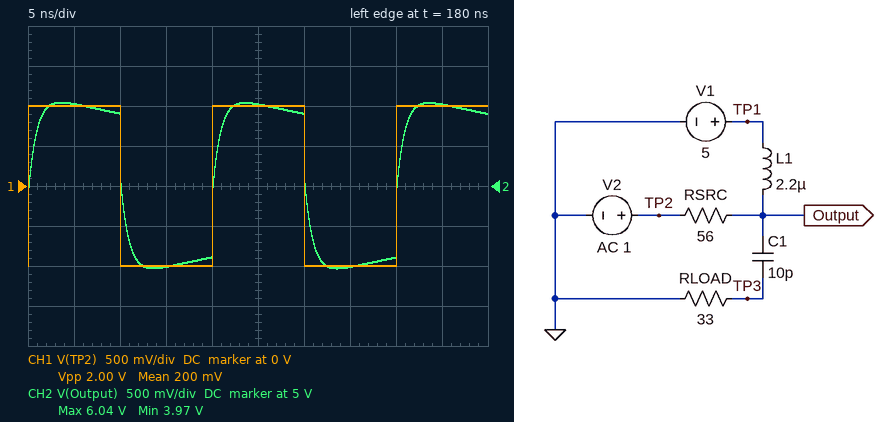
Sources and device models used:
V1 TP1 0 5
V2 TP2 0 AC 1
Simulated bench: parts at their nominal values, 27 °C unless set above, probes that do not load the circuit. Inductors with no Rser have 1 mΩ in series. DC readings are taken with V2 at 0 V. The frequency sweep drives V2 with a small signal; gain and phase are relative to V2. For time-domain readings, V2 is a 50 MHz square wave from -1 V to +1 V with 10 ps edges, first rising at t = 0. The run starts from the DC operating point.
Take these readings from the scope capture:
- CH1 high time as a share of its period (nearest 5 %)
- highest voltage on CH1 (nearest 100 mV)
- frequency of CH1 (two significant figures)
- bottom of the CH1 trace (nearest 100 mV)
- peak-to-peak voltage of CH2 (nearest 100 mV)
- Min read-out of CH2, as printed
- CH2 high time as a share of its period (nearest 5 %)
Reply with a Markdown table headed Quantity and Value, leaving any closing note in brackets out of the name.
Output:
| Quantity | Value |
|---|---|
| CH1 high time as a share of its period | 50 % |
| highest voltage on CH1 | 1.0 V |
| frequency of CH1 | 50 MHz |
| bottom of the CH1 trace | -1.0 V |
| peak-to-peak voltage of CH2 | 2.1 V |
| Min read-out of CH2, as printed | 3.97 V |
| CH2 high time as a share of its period | 50 % |
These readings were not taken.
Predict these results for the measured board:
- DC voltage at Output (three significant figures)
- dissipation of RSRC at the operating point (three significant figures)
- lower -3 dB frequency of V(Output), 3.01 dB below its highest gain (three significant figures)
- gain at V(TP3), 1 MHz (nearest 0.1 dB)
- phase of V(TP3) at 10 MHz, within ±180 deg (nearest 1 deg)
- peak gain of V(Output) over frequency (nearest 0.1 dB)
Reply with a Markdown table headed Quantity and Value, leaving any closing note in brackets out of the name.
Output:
| Quantity | Value |
|---|---|
| DC voltage at Output | 5.00 V |
| dissipation of RSRC at the operating point | 446 mW |
| lower -3 dB frequency of V(Output), 3.01 dB below its highest gain | 3.94 MHz |
| gain at V(TP3), 1 MHz | -66.1 dB |
| phase of V(TP3) at 10 MHz, within ±180 deg | 109 deg |
| peak gain of V(Output) over frequency | -0.1 dB |
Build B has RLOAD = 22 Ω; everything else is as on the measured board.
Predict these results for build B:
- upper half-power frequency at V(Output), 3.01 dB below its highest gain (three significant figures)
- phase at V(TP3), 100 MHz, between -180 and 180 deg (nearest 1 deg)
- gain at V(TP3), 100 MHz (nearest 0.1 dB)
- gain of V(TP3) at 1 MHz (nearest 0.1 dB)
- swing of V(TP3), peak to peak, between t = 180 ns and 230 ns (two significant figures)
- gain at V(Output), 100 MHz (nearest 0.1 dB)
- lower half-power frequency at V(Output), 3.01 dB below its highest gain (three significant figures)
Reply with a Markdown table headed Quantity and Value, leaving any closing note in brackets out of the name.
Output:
| Quantity | Value |
|---|---|
| upper half-power frequency at V(Output), 3.01 dB below its highest gain | 228 MHz |
| phase at V(TP3), 100 MHz, between -180 and 180 deg | 66 deg |
| gain at V(TP3), 100 MHz | -18.0 dB |
| gain of V(TP3) at 1 MHz | -69.6 dB |
| swing of V(TP3), peak to peak, between t = 180 ns and 230 ns | 1.1 V |
| gain at V(Output), 100 MHz | -0.8 dB |
| lower half-power frequency at V(Output), 3.01 dB below its highest gain | 3.96 MHz |
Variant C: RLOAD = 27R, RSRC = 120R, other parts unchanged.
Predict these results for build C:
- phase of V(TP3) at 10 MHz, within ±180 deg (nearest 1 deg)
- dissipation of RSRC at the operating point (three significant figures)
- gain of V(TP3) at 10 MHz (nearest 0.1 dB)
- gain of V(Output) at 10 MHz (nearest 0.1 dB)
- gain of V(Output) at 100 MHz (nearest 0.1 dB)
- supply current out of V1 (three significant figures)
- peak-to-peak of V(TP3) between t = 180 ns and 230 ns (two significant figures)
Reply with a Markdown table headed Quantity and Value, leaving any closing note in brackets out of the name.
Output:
| Quantity | Value |
|---|---|
| phase of V(TP3) at 10 MHz, within ±180 deg | 127 deg |
| dissipation of RSRC at the operating point | 208 mW |
| gain of V(TP3) at 10 MHz | -37.5 dB |
| gain of V(Output) at 10 MHz | -2.1 dB |
| gain of V(Output) at 100 MHz | -2.3 dB |
| supply current out of V1 | 41.7 mA |
| peak-to-peak of V(TP3) between t = 180 ns and 230 ns | 760 mV |
